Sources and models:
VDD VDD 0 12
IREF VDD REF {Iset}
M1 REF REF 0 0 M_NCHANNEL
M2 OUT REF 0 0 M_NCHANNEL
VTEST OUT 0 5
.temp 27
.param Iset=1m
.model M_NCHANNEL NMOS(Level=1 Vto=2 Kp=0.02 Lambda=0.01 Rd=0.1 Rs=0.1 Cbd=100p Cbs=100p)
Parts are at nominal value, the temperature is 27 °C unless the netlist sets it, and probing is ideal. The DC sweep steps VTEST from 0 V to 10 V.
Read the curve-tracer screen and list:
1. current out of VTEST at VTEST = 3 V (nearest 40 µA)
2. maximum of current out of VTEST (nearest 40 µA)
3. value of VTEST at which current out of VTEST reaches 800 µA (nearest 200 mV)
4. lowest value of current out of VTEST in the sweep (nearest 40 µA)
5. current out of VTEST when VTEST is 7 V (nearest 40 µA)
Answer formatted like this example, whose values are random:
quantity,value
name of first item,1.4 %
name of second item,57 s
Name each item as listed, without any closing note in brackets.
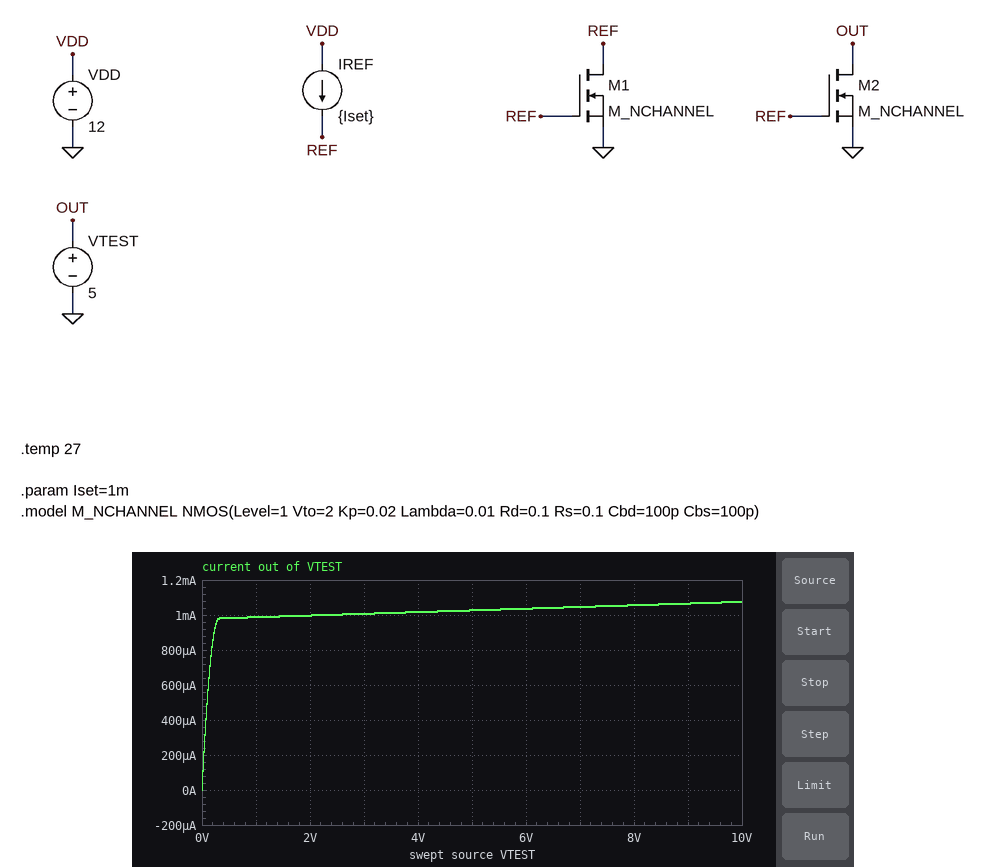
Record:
quantity,value
current out of VTEST at VTEST = 3 V,1.00 mA
maximum of current out of VTEST,1.08 mA
value of VTEST at which current out of VTEST reaches 800 µA,200 mV
lowest value of current out of VTEST in the sweep,0 A
current out of VTEST when VTEST is 7 V,1.04 mA
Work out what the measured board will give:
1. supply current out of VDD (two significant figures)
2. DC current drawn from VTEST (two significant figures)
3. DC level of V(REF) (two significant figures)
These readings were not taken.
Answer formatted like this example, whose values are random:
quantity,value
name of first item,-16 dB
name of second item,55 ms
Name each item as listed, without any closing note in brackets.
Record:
quantity,value
supply current out of VDD,1.0 mA
DC current drawn from VTEST,1.0 mA
DC level of V(REF),2.3 V
